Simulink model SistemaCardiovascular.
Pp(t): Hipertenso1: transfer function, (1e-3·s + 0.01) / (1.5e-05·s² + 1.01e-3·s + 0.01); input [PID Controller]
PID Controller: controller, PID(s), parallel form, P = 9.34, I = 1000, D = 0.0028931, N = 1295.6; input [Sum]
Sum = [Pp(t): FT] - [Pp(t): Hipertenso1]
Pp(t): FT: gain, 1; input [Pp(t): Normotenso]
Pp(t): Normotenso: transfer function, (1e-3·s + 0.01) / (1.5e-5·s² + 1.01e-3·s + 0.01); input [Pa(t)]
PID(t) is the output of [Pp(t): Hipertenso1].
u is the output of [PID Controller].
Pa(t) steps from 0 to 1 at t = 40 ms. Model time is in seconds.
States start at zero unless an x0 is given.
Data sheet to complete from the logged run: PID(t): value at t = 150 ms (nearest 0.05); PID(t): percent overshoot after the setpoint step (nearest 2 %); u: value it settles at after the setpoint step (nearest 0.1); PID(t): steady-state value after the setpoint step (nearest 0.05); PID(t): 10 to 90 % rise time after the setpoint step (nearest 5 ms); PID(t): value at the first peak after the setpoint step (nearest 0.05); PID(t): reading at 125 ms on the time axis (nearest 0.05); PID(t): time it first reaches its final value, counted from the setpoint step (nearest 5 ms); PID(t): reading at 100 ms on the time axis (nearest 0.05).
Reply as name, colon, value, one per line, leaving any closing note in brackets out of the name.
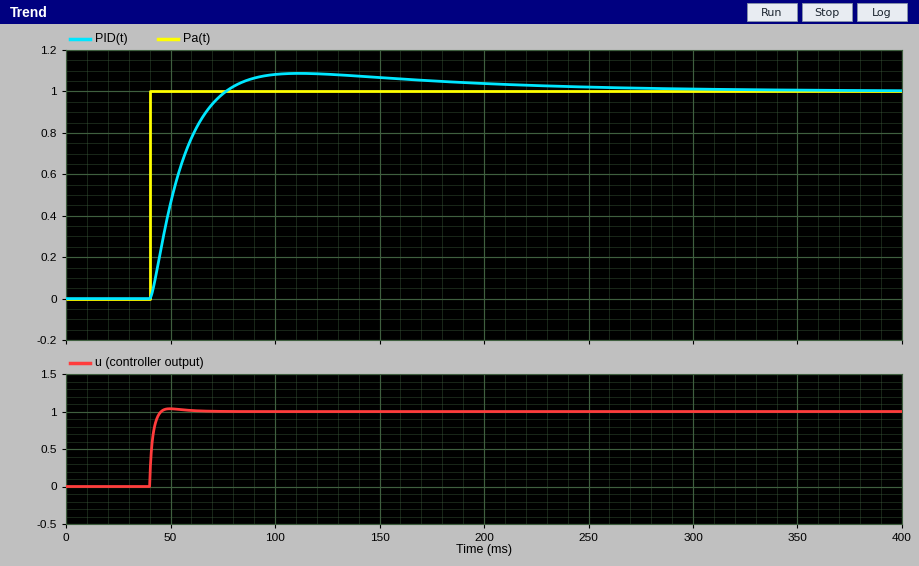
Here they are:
PID(t): value at t = 150 ms: 1.05
PID(t): percent overshoot after the setpoint step: 8 %
u: value it settles at after the setpoint step: 1.0
PID(t): steady-state value after the setpoint step: 1.00
PID(t): 10 to 90 % rise time after the setpoint step: 25 ms
PID(t): value at the first peak after the setpoint step: 1.10
PID(t): reading at 125 ms on the time axis: 1.10
PID(t): time it first reaches its final value, counted from the setpoint step: 35 ms
PID(t): reading at 100 ms on the time axis: 1.10
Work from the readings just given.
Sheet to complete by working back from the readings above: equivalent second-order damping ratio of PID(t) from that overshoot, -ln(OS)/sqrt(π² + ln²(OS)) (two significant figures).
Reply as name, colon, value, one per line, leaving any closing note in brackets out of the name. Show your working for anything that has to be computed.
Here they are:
equivalent second-order damping ratio of PID(t) from that overshoot, -ln(OS)/sqrt(π² + ln²(OS)): ln(0.08) = -2.526; 2.526 / sqrt(9.870 + 6.379) = 0.63
